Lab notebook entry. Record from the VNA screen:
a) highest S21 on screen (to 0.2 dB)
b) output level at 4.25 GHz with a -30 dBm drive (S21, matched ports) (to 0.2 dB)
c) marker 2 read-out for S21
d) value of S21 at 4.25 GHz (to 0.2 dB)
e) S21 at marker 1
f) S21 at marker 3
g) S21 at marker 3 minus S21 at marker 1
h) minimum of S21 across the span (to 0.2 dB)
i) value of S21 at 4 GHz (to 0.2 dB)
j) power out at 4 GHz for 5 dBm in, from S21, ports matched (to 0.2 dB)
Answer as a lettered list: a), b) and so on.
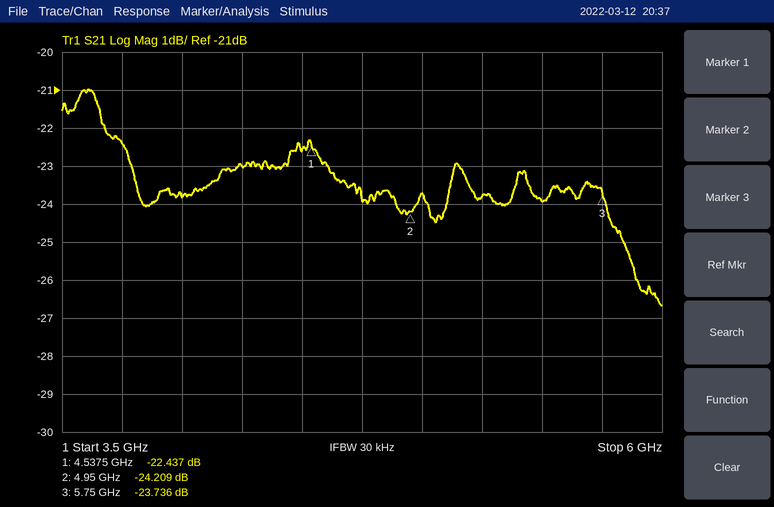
a) -21.0 dB
b) -53.0 dBm
c) -24.209 dB
d) -23.0 dB
e) -22.437 dB
f) -23.736 dB
g) -1.299 dB
h) -26.6 dB
i) -23.8 dB
j) -18.8 dBm
